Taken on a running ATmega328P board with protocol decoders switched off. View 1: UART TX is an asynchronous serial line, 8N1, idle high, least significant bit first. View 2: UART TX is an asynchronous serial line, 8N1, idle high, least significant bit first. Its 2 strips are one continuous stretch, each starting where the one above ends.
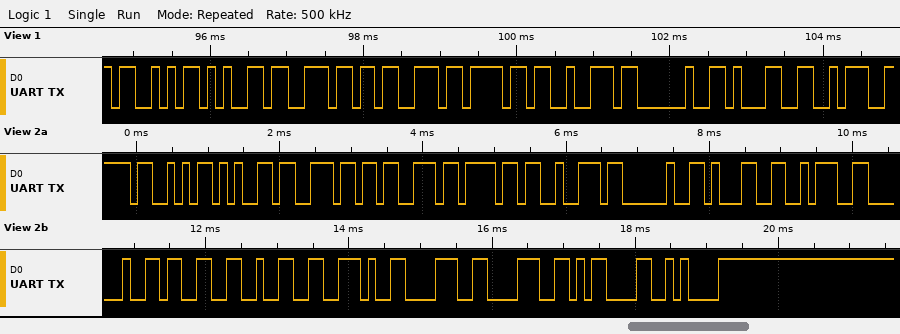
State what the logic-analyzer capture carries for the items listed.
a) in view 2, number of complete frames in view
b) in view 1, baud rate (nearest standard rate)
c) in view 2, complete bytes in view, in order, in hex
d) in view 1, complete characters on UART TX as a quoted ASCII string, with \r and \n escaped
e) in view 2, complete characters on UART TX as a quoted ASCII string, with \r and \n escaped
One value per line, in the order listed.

17
9600 baud
53 65 6E 73 6F 72 20 31 3A 20 33 32 2E 38 38 0D 0A
"Sensor 1:"
"Sensor 1: 32.88\r\n"
